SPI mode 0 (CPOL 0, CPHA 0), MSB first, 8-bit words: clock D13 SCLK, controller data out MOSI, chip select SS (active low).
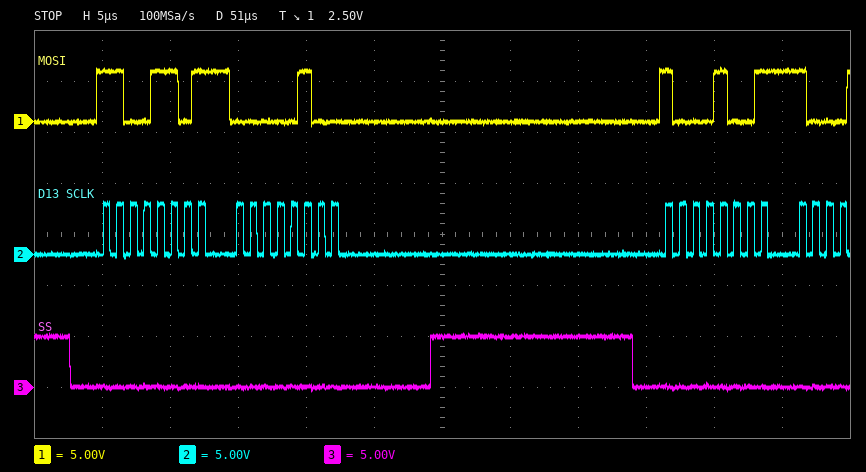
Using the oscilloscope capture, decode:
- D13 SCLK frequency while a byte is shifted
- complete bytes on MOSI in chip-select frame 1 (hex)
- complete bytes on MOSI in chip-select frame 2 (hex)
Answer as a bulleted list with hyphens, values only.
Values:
- 1 MHz
- CD 04
- 89
